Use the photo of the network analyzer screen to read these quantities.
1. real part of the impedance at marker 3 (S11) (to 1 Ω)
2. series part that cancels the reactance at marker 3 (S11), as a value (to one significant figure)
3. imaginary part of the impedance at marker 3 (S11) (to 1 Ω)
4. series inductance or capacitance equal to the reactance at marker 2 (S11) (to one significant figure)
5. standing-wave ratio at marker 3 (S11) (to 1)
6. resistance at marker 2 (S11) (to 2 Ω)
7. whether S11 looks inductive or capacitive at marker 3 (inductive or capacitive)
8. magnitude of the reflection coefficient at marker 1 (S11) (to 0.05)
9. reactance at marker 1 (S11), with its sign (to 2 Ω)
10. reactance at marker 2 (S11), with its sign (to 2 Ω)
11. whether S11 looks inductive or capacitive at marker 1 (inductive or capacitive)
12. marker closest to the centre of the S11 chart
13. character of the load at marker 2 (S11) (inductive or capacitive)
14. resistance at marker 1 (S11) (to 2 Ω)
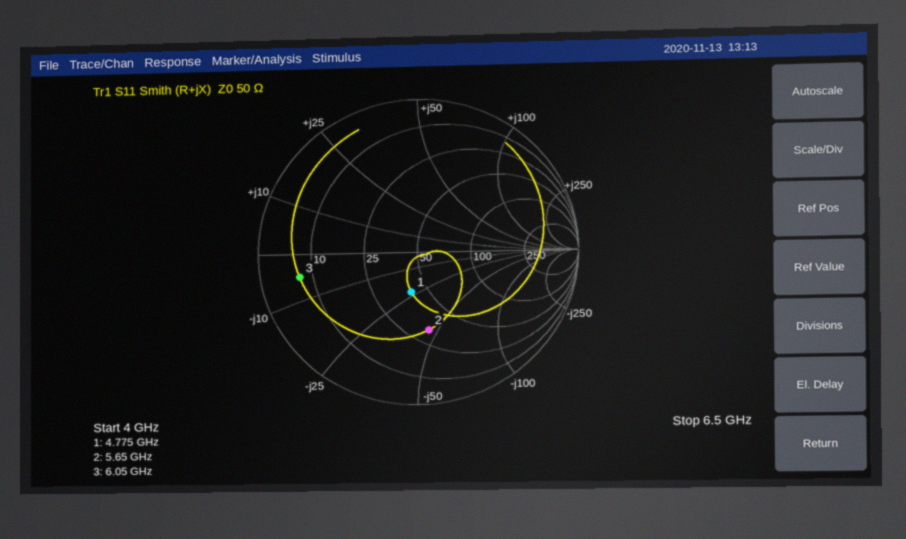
7 Ω
100 pH
-5 Ω
600 fF
7
32 Ω
capacitive
0.25
-22 Ω
-46 Ω
capacitive
marker 1
capacitive
40 Ω
